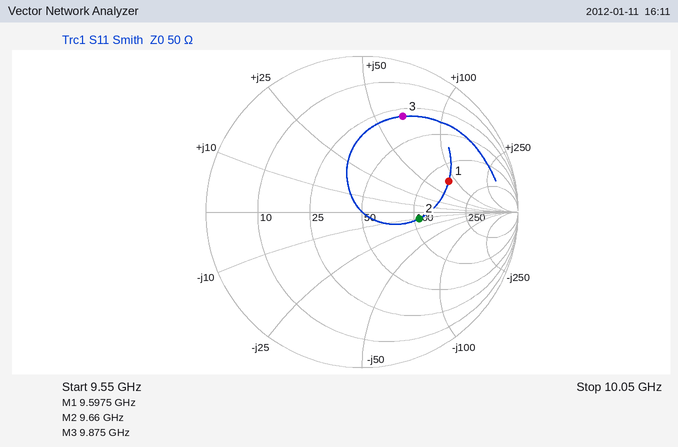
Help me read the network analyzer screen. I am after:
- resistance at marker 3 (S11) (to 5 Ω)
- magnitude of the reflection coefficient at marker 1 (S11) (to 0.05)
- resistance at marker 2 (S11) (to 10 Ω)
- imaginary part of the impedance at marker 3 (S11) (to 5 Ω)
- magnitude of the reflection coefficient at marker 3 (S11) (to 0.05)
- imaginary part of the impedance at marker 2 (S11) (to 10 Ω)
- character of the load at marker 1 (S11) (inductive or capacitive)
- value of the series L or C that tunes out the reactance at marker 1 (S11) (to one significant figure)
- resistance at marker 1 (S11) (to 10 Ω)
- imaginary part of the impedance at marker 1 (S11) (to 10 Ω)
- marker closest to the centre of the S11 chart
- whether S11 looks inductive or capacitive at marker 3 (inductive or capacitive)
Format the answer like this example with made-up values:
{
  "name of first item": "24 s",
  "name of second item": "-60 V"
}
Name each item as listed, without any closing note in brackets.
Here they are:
{
  "resistance at marker 3 (S11)": "30 Ω",
  "magnitude of the reflection coefficient at marker 1 (S11)": "0.60",
  "resistance at marker 2 (S11)": "110 Ω",
  "imaginary part of the impedance at marker 3 (S11)": "+65 Ω",
  "magnitude of the reflection coefficient at marker 3 (S11)": "0.65",
  "imaginary part of the impedance at marker 2 (S11)": "-10 Ω",
  "character of the load at marker 1 (S11)": "inductive",
  "value of the series L or C that tunes out the reactance at marker 1 (S11)": "200 fF",
  "resistance at marker 1 (S11)": "140 Ω",
  "imaginary part of the impedance at marker 1 (S11)": "+80 Ω",
  "marker closest to the centre of the S11 chart": "marker 2",
  "whether S11 looks inductive or capacitive at marker 3": "inductive"
}
